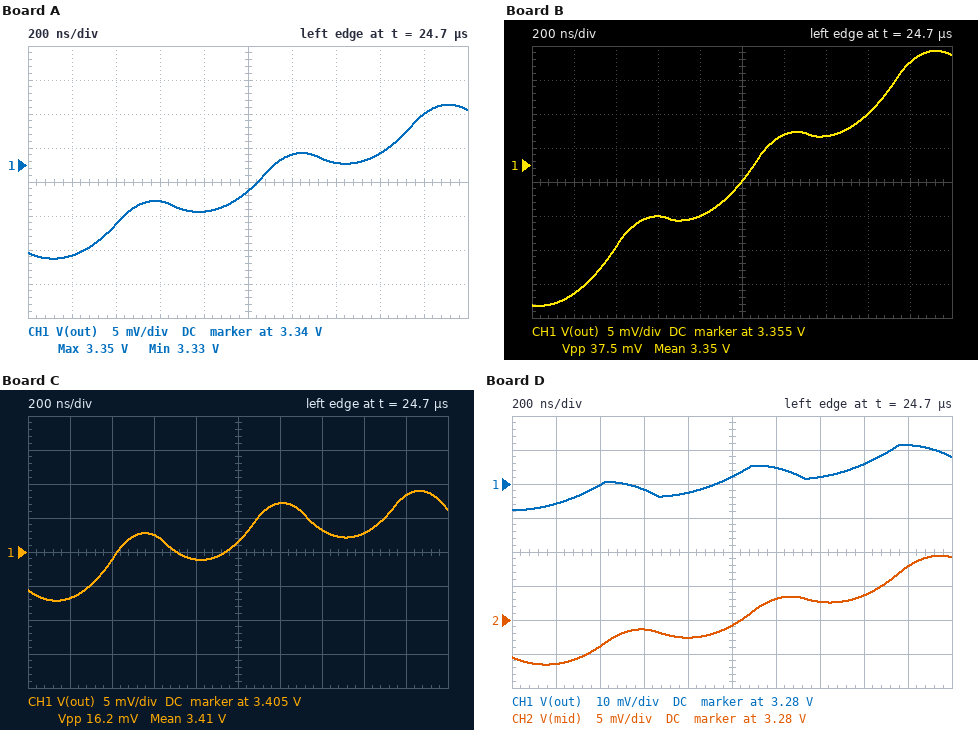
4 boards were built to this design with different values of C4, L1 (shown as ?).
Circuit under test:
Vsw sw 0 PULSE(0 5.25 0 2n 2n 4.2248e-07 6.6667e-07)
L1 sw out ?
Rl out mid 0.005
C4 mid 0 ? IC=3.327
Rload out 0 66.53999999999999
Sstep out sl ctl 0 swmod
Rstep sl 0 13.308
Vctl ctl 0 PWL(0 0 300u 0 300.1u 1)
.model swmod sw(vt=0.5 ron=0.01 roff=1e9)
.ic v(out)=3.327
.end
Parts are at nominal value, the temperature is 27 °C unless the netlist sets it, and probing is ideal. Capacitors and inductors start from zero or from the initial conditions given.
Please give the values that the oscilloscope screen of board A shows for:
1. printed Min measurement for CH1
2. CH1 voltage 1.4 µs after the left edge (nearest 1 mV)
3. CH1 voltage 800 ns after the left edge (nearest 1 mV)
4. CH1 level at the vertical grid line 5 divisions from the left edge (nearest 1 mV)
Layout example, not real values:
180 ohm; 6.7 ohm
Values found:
3.33 V; 3.340 V; 3.333 V; 3.336 V
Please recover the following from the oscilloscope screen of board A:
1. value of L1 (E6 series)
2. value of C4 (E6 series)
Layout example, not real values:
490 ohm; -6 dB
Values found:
4.7 µH; 3.3 µF
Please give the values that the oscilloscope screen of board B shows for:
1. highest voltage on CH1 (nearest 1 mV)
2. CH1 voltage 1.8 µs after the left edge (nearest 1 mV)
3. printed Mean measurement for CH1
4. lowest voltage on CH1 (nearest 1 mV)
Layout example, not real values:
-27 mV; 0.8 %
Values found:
3.372 V; 3.370 V; 3.35 V; 3.334 V
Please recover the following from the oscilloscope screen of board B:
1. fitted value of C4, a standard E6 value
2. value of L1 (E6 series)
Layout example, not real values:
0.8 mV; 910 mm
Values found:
6.8 µF; 2.2 µH
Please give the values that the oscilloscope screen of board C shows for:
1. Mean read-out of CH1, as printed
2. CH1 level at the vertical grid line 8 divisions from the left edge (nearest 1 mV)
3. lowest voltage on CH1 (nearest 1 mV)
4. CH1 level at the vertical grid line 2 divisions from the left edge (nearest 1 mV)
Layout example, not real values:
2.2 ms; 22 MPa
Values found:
3.41 V; 3.408 V; 3.398 V; 3.404 V
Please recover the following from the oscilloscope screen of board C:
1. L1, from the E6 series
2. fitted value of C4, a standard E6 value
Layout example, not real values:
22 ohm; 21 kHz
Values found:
3.3 µH; 3.3 µF
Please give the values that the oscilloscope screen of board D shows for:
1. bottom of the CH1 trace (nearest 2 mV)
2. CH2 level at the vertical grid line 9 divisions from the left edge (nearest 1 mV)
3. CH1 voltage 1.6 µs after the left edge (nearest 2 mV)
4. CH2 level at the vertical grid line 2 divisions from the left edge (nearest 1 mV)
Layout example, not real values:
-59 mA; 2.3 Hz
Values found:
3.272 V; 3.288 V; 3.286 V; 3.276 V
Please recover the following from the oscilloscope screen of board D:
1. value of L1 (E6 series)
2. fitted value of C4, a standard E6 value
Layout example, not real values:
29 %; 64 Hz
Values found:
680 nH; 33 µF
